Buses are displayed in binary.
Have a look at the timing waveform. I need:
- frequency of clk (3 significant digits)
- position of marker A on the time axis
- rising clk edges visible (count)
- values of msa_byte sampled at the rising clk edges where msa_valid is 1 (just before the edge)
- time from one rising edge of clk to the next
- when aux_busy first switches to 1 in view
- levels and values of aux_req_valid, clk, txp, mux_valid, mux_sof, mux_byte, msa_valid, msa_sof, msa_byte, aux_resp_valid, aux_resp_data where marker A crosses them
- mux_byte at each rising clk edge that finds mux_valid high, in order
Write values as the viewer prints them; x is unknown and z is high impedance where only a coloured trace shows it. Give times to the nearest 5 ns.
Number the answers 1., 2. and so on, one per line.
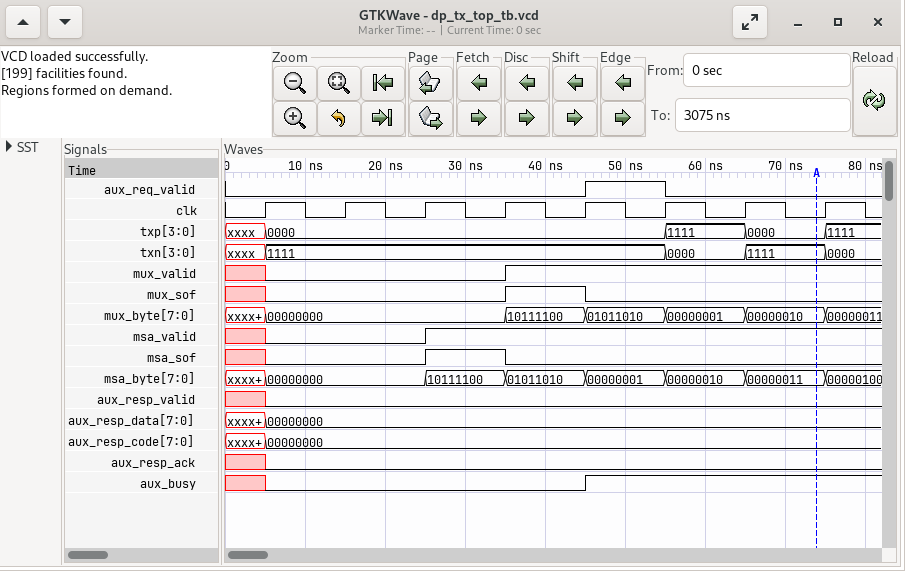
1. 100 MHz
2. 75 ns
3. 8
4. 10111100, 01011010, 00000001, 00000010, 00000011
5. 10 ns
6. 45 ns
7. aux_req_valid=0, clk=0, txp=0000, mux_valid=1, mux_sof=0, mux_byte=00000010, msa_valid=1, msa_sof=0, msa_byte=00000011, aux_resp_valid=0, aux_resp_data=00000000
8. 10111100, 01011010, 00000001, 00000010
